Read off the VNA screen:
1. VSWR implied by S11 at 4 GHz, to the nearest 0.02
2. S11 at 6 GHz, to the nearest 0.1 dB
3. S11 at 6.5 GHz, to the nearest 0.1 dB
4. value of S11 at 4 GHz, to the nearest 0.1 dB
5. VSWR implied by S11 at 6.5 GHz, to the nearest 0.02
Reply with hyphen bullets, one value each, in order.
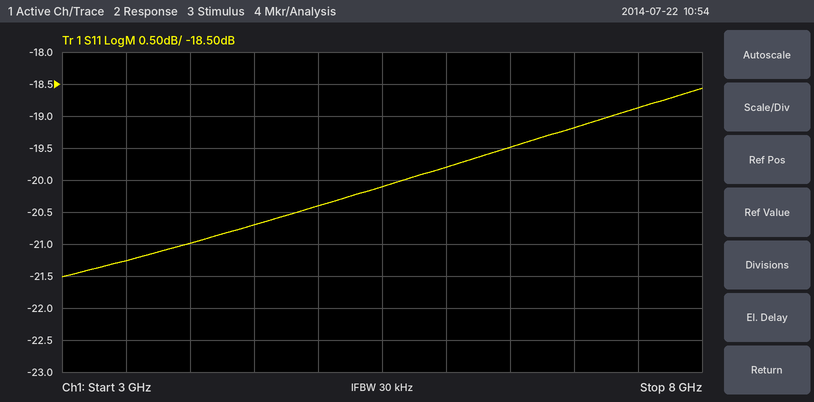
- 1.20
- -19.8 dB
- -19.5 dB
- -21.0 dB
- 1.24
